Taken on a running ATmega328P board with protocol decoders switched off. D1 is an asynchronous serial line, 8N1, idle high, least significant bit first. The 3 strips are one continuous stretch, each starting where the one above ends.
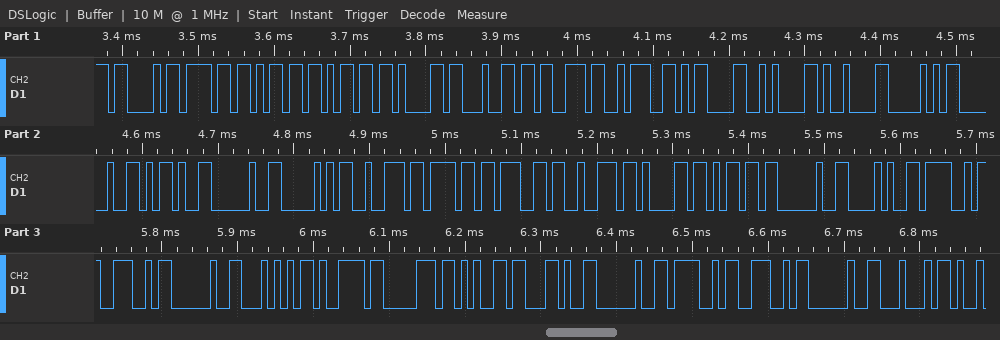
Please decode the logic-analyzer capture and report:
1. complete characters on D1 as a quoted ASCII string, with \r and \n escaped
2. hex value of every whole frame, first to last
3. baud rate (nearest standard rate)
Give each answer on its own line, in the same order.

"Commads:\r\n\tP - Program (ON Type, ON D"
43 6F 6D 6D 61 64 73 3A 0D 0A 09 50 20 2D 20 50 72 6F 67 72 61 6D 20 28 4F 4E 20 54 79 70 65 2C 20 4F 4E 20 44
115200 baud
